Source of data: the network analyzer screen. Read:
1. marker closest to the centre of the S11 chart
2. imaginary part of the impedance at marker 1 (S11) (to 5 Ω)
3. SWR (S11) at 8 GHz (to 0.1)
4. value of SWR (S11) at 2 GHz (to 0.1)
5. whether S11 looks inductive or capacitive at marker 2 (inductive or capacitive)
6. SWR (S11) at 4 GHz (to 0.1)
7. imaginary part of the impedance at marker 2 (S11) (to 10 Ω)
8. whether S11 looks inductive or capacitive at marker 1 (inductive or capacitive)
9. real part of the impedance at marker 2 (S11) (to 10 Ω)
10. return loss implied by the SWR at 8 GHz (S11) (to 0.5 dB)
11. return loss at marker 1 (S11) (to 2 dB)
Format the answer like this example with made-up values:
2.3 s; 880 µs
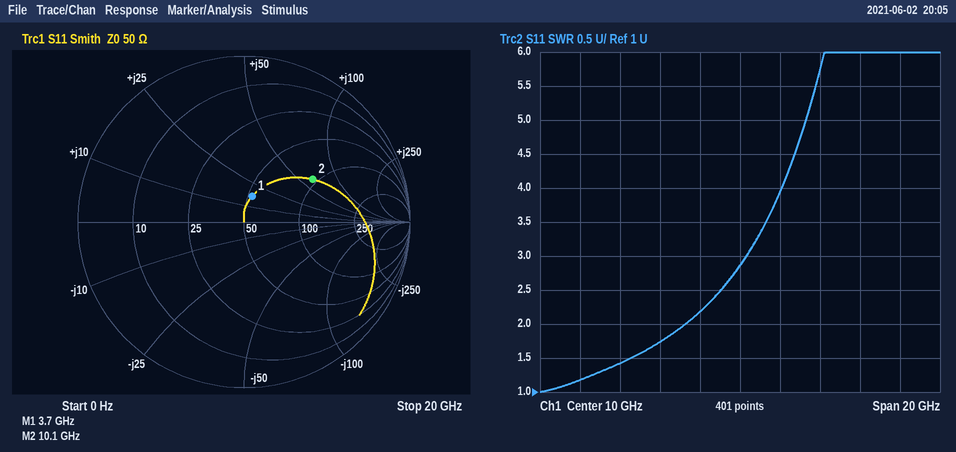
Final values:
marker 1; +15 Ω; 2.2; 1.2; inductive; 1.4; +60 Ω; inductive; 90 Ω; 8.5 dB; 16 dB
